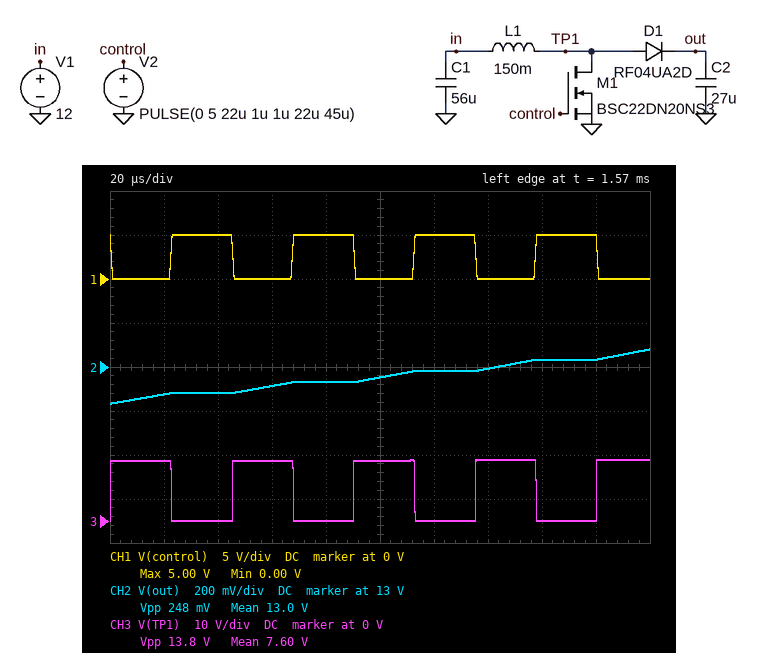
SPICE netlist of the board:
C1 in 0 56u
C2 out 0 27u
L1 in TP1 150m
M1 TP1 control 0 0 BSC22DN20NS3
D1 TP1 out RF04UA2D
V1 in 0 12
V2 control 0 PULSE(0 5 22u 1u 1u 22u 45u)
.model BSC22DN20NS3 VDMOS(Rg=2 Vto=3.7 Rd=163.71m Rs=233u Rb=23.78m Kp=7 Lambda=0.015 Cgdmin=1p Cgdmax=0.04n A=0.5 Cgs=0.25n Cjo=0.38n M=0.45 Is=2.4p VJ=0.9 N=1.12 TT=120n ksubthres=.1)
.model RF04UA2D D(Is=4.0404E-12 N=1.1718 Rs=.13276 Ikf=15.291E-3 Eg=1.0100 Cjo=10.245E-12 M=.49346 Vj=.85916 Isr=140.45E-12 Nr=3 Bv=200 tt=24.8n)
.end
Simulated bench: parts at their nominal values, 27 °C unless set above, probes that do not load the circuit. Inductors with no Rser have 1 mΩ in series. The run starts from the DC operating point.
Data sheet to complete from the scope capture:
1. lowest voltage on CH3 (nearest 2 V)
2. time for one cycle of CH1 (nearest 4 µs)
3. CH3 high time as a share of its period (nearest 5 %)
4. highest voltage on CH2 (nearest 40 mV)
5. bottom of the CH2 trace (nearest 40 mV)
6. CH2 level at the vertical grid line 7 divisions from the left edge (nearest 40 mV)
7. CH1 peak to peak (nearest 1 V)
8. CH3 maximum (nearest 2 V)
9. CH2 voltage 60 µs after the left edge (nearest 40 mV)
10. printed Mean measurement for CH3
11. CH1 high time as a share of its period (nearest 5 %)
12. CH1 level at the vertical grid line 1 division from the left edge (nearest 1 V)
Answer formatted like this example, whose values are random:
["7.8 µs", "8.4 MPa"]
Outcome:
["0 V", "44 µs", "50 %", "13.08 V", "12.84 V", "13.00 V", "5 V", "14 V", "12.92 V", "7.60 V", "50 %", "0 V"]
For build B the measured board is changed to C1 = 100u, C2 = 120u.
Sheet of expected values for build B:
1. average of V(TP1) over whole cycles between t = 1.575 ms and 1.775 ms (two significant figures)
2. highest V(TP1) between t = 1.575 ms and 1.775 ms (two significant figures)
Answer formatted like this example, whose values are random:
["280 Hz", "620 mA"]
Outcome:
["6.5 V", "13 V"]
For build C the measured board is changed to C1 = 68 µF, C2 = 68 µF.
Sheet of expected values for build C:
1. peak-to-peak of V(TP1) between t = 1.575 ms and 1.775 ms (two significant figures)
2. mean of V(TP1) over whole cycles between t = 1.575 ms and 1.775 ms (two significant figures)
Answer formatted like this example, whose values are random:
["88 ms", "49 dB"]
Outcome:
["13 V", "6.6 V"]
